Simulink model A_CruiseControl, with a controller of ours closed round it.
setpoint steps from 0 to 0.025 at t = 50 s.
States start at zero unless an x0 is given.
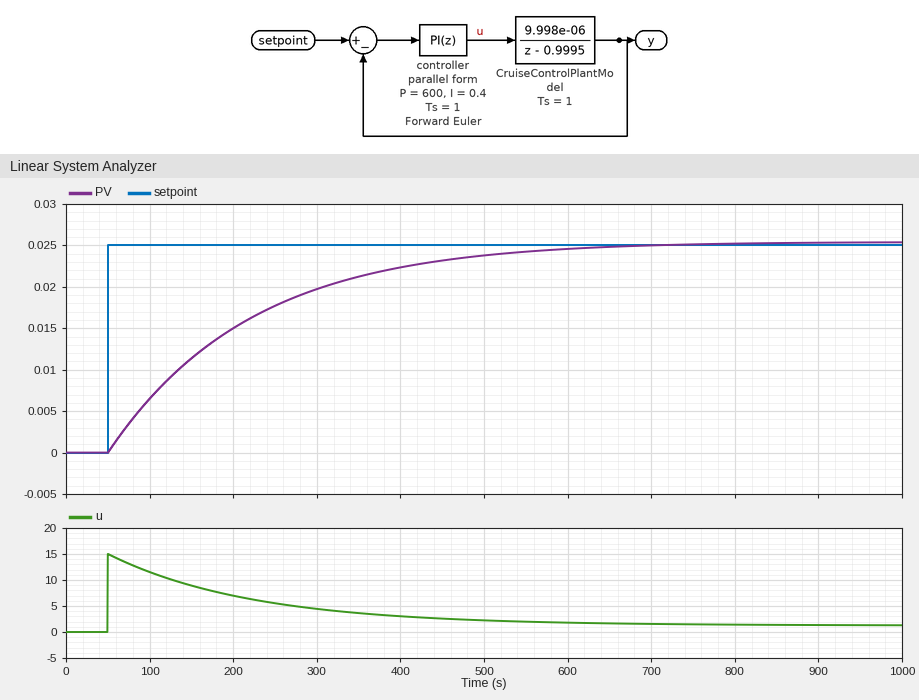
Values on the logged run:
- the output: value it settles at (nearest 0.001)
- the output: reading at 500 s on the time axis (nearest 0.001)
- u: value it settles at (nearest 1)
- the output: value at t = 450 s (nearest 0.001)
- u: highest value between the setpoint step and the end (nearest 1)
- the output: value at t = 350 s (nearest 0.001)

0.025
0.024
1
0.023
15
0.021
